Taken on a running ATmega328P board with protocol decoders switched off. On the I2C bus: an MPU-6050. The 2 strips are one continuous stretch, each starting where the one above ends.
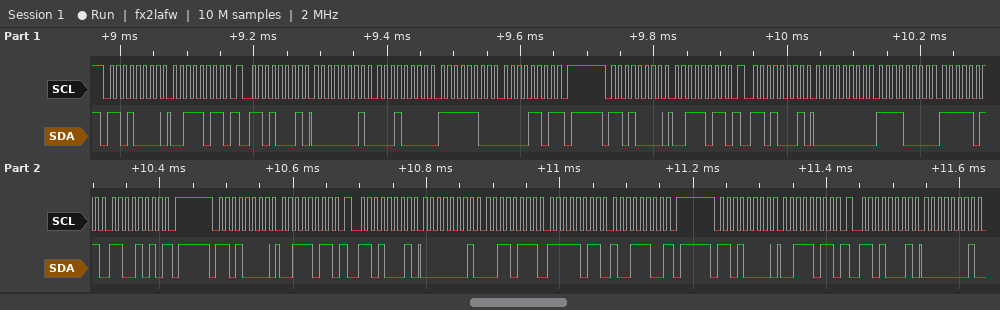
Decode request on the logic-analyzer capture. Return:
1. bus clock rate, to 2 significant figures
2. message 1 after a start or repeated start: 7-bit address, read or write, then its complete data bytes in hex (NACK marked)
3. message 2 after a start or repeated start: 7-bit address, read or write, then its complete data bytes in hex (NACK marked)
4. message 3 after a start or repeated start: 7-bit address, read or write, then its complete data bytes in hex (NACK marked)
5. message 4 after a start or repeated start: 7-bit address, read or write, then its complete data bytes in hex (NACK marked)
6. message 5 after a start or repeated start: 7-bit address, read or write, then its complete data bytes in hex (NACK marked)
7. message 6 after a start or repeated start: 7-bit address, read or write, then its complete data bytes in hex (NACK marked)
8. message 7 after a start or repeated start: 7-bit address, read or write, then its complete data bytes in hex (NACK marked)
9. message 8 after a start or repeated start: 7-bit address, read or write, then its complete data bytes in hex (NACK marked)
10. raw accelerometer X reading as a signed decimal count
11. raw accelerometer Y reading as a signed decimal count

100 kHz
0x68 write: 3B
0x68 read: 01 10 FC 0D NACK
0x68 write: 3B
0x68 read: 00 F0 FB CA NACK
0x68 write: 3B
0x68 read: 01 37 FB 9C NACK
0x68 write: 3B
0x68 read: 01
272
-1011
